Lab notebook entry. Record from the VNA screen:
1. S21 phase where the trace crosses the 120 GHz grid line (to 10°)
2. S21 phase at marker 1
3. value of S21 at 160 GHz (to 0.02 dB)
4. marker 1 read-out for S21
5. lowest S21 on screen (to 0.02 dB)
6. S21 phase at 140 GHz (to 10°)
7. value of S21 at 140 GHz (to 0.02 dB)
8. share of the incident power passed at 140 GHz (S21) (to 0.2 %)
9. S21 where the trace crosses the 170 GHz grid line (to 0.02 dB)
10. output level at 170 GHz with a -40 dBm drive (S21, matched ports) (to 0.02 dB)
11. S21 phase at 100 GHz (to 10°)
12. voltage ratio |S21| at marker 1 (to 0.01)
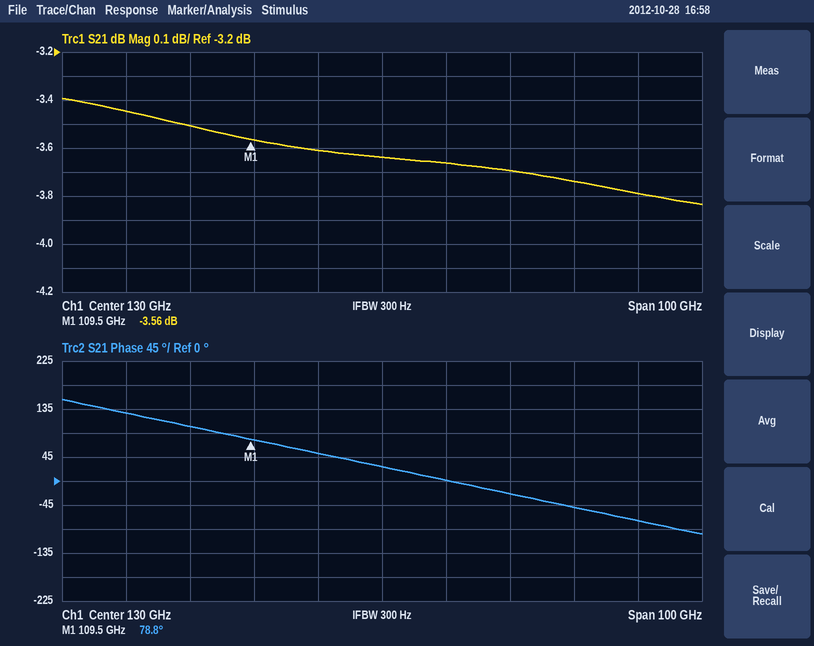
50°
78.8°
-3.74 dB
-3.56 dB
-3.84 dB
0°
-3.66 dB
43.0 %
-3.78 dB
-43.78 dBm
100°
0.66
